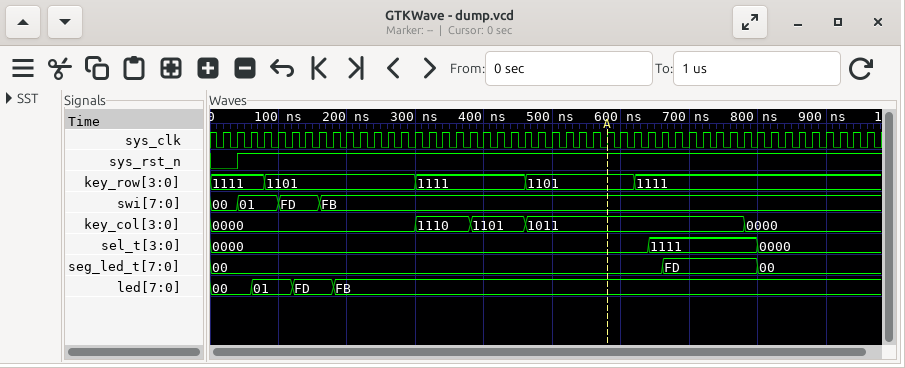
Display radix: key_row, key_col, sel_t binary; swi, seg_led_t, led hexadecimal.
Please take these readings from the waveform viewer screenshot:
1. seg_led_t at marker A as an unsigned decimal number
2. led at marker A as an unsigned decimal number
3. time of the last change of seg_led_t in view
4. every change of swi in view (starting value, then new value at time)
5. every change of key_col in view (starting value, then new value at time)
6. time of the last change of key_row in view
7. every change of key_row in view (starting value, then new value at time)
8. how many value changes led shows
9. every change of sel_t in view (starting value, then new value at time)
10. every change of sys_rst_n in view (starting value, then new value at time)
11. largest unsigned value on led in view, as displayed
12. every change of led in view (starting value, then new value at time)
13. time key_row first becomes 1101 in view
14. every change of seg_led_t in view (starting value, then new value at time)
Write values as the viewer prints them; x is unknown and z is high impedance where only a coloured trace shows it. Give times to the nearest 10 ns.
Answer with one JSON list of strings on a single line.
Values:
["0", "251", "800 ns", "00, 01 at 40 ns, FD at 100 ns, FB at 160 ns", "0000, 1110 at 300 ns, 1101 at 380 ns, 1011 at 460 ns, 0000 at 780 ns", "620 ns", "1111, 1101 at 80 ns, 1111 at 300 ns, 1101 at 460 ns, 1111 at 620 ns", "3", "0000, 1111 at 640 ns, 0000 at 800 ns", "0, 1 at 40 ns", "FD", "00, 01 at 60 ns, FD at 120 ns, FB at 180 ns", "80 ns", "00, FD at 660 ns, 00 at 800 ns"]
